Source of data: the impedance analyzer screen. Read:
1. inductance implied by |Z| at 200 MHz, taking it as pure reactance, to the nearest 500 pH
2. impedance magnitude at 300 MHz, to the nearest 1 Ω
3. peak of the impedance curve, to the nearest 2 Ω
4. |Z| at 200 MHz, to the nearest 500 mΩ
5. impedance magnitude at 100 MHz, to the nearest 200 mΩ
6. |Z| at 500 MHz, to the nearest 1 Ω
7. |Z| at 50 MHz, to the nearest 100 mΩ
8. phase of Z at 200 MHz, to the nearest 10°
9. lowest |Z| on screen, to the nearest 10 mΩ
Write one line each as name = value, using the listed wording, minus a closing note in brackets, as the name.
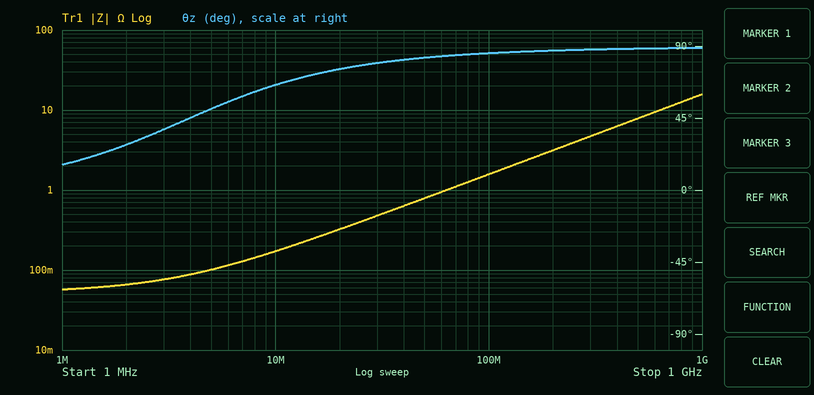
inductance implied by |Z| at 200 MHz, taking it as pure reactance, to the nearest 500 pH = 2.5 nH
impedance magnitude at 300 MHz, to the nearest 1 Ω = 5 Ω
peak of the impedance curve, to the nearest 2 Ω = 16 Ω
|Z| at 200 MHz, to the nearest 500 mΩ = 3.0 Ω
impedance magnitude at 100 MHz, to the nearest 200 mΩ = 1.6 Ω
|Z| at 500 MHz, to the nearest 1 Ω = 8 Ω
|Z| at 50 MHz, to the nearest 100 mΩ = 800 mΩ
phase of Z at 200 MHz, to the nearest 10° = 90°
lowest |Z| on screen, to the nearest 10 mΩ = 60 mΩ
